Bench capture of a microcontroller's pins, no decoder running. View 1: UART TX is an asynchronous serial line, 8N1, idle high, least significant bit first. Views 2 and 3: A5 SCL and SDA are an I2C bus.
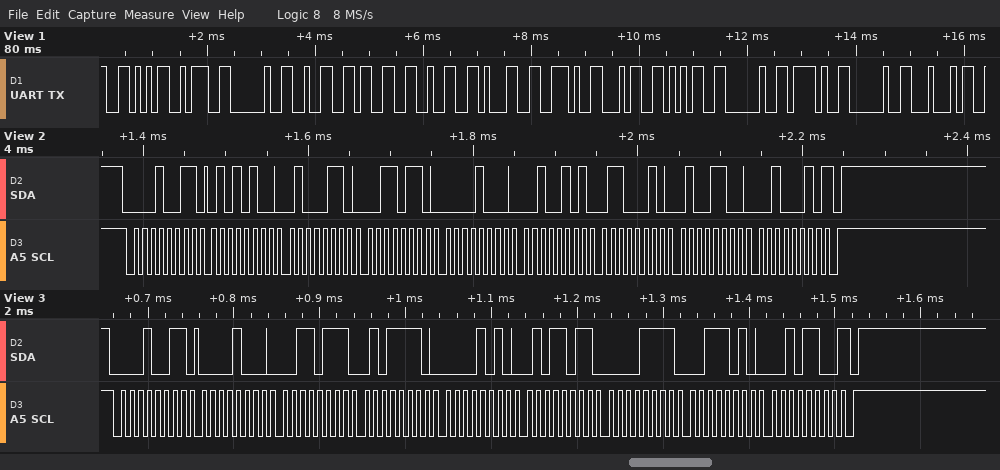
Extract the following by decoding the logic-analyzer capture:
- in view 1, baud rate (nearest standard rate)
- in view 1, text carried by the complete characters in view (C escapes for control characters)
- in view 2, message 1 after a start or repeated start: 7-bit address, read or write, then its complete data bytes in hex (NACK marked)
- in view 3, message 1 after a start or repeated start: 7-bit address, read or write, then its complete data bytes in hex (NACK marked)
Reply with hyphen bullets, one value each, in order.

- 9600 baud
- "V: 2321.45 / D"
- 0x09 read: 54 46 36 08 25 62 4C 22 NACK
- 0x09 read: 08 37 5E 0A 5B 0F 3A 2C NACK
